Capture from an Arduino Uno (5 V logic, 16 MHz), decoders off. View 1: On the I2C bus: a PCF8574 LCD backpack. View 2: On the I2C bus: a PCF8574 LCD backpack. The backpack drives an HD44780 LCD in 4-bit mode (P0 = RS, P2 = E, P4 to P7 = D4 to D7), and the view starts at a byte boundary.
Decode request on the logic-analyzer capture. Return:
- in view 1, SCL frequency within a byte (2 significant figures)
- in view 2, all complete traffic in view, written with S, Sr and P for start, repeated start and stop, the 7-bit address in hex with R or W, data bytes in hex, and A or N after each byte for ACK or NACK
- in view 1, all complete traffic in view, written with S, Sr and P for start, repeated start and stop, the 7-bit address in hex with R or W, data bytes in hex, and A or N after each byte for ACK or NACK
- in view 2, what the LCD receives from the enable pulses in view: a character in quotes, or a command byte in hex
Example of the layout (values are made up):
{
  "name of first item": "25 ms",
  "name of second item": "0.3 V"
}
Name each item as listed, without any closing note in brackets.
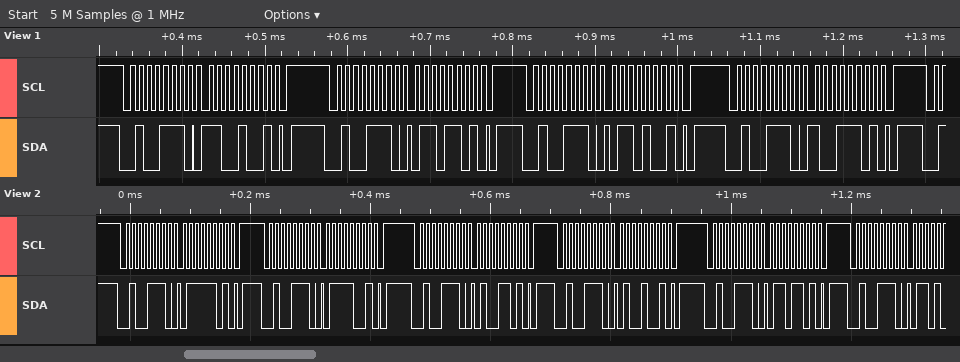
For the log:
{
  "in view 1, SCL frequency within a byte": "100 kHz",
  "in view 2, all complete traffic in view, written with S, Sr and P for start, repeated start and stop, the 7-bit address in hex with R or W, data bytes in hex, and A or N after each byte for ACK or NACK": "S 27W A 7D A P S 27W A 79 A P S 27W A 4D A P S 27W A 49 A P S 27W A 6D A P S 27W A",
  "in view 1, all complete traffic in view, written with S, Sr and P for start, repeated start and stop, the 7-bit address in hex with R or W, data bytes in hex, and A or N after each byte for ACK or NACK": "S 27W A C9 A P S 27W A 6D A P S 27W A 69 A P S 27W A 9D A P",
  "in view 2, what the LCD receives from the enable pulses in view: a character in quotes, or a command byte in hex": "'t'"
}
